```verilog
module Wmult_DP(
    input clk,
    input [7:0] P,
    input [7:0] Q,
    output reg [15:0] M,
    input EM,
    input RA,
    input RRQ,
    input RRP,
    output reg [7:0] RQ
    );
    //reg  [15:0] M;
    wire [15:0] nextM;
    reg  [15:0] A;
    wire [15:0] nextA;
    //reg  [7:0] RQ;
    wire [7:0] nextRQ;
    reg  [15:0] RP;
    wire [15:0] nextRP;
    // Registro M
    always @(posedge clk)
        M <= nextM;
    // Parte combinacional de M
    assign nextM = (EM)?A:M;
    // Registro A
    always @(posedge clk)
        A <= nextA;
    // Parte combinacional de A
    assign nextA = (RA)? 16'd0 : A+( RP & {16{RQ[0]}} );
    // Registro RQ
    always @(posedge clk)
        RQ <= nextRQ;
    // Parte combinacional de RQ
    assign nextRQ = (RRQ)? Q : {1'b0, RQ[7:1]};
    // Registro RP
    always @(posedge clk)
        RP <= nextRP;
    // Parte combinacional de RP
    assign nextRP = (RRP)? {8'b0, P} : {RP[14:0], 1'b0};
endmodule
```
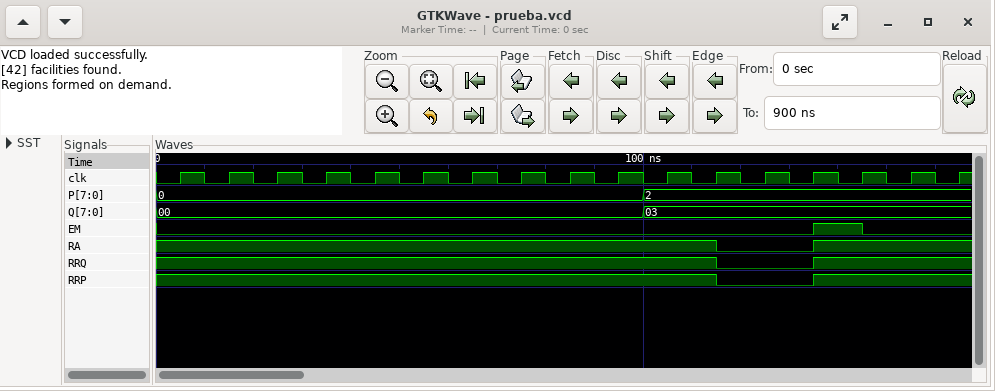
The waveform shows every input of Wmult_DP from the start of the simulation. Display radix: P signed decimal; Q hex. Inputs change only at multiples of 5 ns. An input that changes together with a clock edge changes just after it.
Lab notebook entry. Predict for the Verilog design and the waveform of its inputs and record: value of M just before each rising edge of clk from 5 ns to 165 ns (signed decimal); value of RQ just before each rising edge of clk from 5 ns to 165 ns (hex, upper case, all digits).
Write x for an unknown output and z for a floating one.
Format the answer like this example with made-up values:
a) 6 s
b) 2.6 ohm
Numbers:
a) x, x, x, x, x, x, x, x, x, x, x, x, x, x, x, 6, 6
b) x, 00, 00, 00, 00, 00, 00, 00, 00, 00, 00, 03, 03, 01, 00, 03, 03
